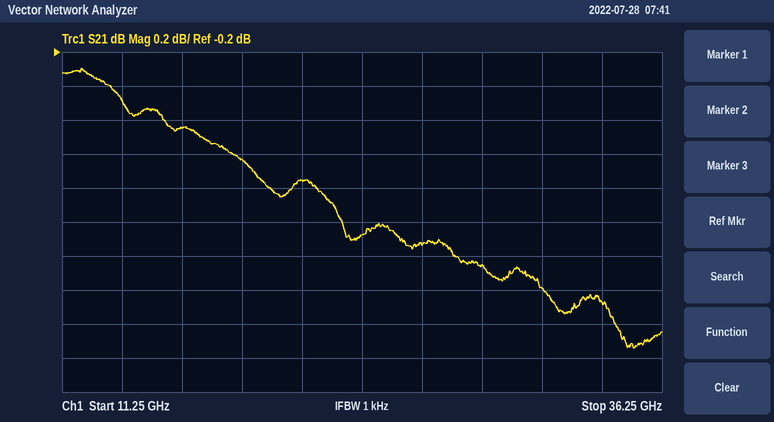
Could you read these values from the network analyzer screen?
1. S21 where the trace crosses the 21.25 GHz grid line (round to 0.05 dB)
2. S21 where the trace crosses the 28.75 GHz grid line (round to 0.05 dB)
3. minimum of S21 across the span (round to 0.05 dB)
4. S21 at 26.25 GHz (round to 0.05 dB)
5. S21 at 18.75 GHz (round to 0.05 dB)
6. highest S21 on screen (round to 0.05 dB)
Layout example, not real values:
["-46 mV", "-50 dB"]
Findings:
["-0.95 dB", "-1.45 dB", "-1.95 dB", "-1.35 dB", "-0.85 dB", "-0.30 dB"]
